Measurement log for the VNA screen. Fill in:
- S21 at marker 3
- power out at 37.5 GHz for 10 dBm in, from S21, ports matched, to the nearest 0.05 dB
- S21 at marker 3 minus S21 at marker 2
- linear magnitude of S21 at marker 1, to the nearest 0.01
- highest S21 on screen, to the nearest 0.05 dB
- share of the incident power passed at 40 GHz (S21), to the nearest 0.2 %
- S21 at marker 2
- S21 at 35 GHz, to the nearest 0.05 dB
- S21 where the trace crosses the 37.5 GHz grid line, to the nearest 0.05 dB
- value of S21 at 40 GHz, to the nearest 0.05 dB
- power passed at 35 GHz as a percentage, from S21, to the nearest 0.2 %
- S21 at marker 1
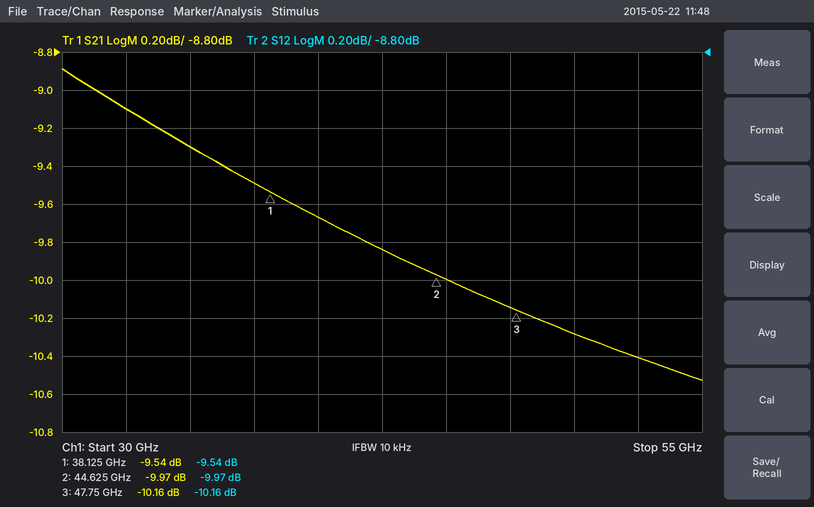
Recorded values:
-10.16 dB
0.50 dBm
-0.19 dB
0.33
-8.90 dB
10.8 %
-9.97 dB
-9.30 dB
-9.50 dB
-9.65 dB
11.8 %
-9.54 dB
